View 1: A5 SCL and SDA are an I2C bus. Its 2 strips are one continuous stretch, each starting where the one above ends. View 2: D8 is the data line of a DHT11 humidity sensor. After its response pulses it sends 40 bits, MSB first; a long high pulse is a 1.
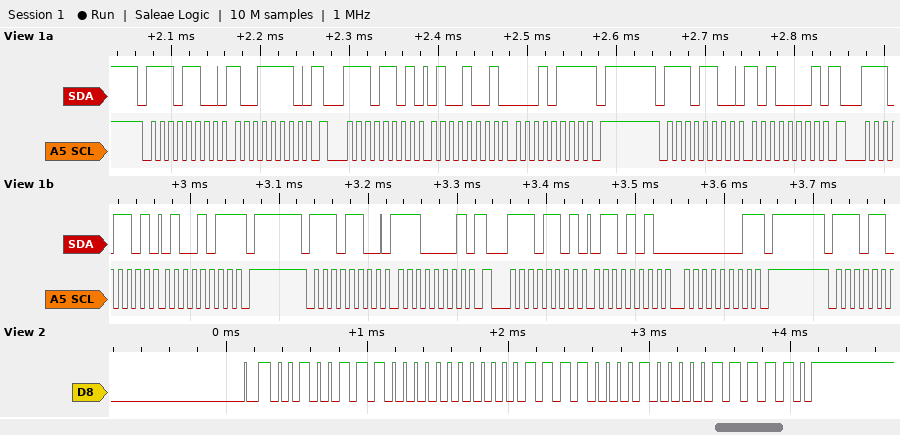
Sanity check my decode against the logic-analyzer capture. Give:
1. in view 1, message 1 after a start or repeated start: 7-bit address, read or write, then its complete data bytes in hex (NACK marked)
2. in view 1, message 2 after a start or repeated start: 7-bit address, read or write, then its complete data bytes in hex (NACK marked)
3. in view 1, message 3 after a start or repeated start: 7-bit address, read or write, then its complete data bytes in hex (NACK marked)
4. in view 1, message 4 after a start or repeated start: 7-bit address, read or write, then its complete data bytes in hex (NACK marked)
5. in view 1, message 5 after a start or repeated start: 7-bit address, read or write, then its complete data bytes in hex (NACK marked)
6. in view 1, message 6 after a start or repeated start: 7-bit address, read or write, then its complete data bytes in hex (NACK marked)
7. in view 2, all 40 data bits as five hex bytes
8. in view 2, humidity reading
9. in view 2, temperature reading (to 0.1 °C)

0x76 write: 9E
0x76 read: 49 17 NACK
0x76 write: A1
0x76 read: 4B NACK
0x76 write: E1
0x76 read: 6A 01 NACK
27 00 0F 08 3E
39 %
15.8 °C
